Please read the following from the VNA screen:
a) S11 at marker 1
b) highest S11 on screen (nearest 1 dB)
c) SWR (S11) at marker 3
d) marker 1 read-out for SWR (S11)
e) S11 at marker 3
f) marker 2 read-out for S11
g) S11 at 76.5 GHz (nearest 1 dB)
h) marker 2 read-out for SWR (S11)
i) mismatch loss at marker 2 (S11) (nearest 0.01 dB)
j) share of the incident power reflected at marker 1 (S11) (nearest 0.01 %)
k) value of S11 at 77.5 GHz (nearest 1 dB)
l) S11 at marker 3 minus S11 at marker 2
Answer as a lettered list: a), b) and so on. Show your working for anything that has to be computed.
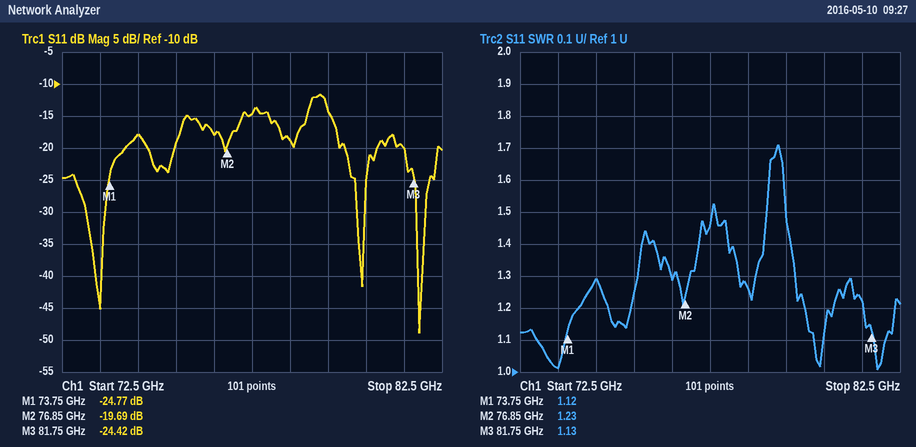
a) -24.77 dB
b) -12 dB
c) 1.13
d) 1.12
e) -24.42 dB
f) -19.69 dB
g) -18 dB
h) 1.23
i) −10 log10(1 − 10^(-19.69/10)) ≈ 0.05 dB
j) 10^(-24.77/10) ≈ 0.33 %
k) -15 dB
l) -24.42 − (-19.69) = -4.73 dB
